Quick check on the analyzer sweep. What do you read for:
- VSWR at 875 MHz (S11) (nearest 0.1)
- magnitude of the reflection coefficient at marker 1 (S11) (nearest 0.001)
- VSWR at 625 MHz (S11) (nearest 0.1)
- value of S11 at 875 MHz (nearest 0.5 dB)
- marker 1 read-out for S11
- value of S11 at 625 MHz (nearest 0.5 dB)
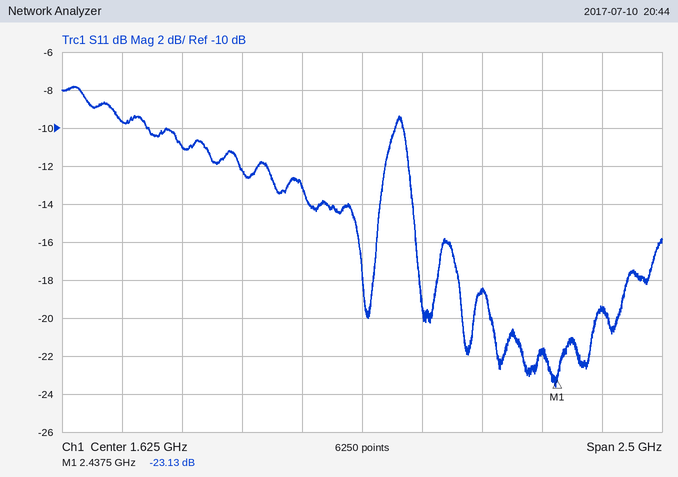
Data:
1.8
0.070
2.0
-11.0 dB
-23.13 dB
-9.5 dB
